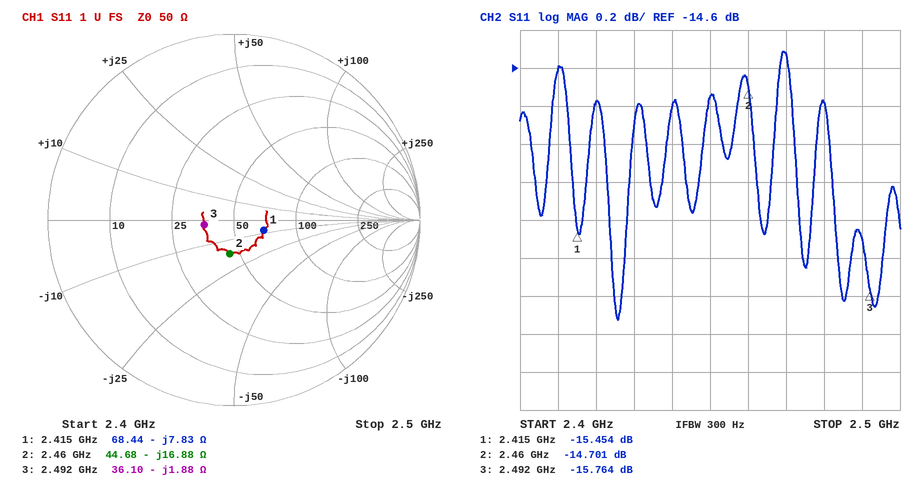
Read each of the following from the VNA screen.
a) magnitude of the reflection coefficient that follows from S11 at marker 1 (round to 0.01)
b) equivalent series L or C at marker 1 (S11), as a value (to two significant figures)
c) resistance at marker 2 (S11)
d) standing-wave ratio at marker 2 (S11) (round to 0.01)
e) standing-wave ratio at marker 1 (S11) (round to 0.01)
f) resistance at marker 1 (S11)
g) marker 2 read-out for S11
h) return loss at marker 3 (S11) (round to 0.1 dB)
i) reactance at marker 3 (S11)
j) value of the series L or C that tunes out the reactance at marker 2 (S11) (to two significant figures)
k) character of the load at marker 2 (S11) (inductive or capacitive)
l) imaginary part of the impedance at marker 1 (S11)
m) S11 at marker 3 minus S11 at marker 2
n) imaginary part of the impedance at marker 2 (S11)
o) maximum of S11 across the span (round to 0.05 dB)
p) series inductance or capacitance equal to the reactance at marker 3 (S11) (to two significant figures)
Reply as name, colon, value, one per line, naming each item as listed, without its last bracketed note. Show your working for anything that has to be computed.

magnitude of the reflection coefficient that follows from S11 at marker 1: 10^(-15.454/20) ≈ 0.17
equivalent series L or C at marker 1 (S11), as a value: C = 1/(2π × 2.415 GHz × 7.83 Ω) ≈ 8.4 pF
resistance at marker 2: 44.68 Ω
standing-wave ratio at marker 2 (S11): 1.45
standing-wave ratio at marker 1 (S11): 1.41
resistance at marker 1: 68.44 Ω
marker 2 read-out for S11: -14.701 dB
return loss at marker 3 (S11): 15.8 dB
reactance at marker 3: -1.88 Ω
value of the series L or C that tunes out the reactance at marker 2 (S11): L = 16.88 Ω/(2π × 2.46 GHz) ≈ 1.1 nH
character of the load at marker 2 (S11): capacitive
imaginary part of the impedance at marker 1: -7.83 Ω
S11 at marker 3 minus S11 at marker 2: -15.764 − (-14.701) = -1.063 dB
imaginary part of the impedance at marker 2: -16.88 Ω
maximum of S11 across the span: -14.50 dB
series inductance or capacitance equal to the reactance at marker 3 (S11): C = 1/(2π × 2.492 GHz × 1.88 Ω) ≈ 34 pF
